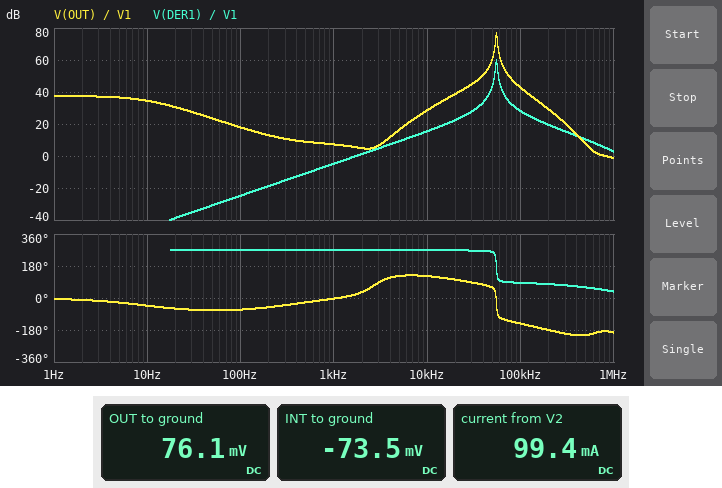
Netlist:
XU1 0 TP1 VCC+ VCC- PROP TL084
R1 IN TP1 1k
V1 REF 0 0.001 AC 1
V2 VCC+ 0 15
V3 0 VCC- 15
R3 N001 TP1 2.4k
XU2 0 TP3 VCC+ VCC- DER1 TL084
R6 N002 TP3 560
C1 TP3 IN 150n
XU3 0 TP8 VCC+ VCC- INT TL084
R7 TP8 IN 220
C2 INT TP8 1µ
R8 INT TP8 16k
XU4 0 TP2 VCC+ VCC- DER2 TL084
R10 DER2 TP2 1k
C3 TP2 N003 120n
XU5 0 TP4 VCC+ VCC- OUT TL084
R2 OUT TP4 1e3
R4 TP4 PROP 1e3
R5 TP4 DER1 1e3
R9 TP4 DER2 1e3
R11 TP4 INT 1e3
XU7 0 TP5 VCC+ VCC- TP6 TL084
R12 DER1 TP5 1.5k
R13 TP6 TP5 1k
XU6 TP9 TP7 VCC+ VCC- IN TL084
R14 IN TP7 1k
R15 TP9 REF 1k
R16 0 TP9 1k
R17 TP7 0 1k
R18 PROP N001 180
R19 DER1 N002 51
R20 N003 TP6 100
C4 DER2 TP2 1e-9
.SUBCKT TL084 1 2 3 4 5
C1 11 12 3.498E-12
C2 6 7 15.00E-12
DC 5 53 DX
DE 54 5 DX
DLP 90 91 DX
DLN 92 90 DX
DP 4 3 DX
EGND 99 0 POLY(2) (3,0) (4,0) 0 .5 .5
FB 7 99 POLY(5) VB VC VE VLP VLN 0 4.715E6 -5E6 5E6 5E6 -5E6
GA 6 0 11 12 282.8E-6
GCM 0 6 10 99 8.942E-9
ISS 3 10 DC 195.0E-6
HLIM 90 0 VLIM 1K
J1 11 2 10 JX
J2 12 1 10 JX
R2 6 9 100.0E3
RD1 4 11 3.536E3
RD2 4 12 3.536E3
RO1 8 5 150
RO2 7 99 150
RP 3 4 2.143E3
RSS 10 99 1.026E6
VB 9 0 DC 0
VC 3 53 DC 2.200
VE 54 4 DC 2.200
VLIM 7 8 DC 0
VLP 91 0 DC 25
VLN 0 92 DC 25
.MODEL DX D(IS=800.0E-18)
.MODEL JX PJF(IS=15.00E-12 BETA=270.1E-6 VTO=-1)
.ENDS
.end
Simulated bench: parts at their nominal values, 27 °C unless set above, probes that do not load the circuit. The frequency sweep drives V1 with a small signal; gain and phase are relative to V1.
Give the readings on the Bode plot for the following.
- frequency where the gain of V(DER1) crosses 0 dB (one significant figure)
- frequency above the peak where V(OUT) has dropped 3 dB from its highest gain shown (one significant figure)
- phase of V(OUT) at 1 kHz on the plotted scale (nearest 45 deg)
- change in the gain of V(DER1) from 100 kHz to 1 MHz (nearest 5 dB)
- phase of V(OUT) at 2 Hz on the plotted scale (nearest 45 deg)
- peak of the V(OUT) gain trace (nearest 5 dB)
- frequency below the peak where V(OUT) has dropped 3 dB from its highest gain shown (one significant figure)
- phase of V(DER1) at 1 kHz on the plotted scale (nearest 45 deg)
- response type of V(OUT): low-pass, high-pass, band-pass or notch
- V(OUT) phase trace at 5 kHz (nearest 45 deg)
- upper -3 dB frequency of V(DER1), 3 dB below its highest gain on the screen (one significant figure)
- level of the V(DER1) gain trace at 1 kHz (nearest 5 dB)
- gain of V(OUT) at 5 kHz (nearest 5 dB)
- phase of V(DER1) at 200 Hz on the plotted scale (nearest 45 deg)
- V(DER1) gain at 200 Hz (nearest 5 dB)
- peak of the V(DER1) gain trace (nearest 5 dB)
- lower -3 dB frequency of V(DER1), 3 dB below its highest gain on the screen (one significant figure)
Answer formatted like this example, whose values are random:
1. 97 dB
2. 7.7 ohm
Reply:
1. 2 kHz
2. 60 kHz
3. 0 deg
4. -25 dB
5. 0 deg
6. 75 dB
7. 50 kHz
8. 270 deg
9. band-pass
10. 135 deg
11. 60 kHz
12. -5 dB
13. 15 dB
14. 270 deg
15. -20 dB
16. 60 dB
17. 50 kHz
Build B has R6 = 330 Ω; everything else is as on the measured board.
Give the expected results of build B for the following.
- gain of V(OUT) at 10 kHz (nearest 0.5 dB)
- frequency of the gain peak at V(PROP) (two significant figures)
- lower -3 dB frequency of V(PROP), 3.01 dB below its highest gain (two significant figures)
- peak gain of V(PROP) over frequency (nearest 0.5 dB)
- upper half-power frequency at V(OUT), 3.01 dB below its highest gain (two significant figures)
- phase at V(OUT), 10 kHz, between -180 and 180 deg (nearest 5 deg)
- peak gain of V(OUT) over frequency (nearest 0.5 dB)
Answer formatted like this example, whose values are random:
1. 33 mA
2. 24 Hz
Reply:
1. 24.0 dB
2. 63 kHz
3. 62 kHz
4. 27.0 dB
5. 64 kHz
6. 120 deg
7. 72.0 dB
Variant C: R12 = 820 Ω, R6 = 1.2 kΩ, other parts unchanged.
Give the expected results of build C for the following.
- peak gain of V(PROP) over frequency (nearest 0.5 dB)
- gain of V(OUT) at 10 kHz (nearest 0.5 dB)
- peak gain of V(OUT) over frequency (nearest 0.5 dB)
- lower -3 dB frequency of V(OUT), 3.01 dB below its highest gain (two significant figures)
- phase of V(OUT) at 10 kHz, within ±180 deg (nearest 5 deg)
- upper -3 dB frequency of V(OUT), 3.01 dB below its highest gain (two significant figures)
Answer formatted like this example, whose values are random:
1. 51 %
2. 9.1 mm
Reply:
1. 21.0 dB
2. 40.0 dB
3. 85.0 dB
4. 41 kHz
5. 130 deg
6. 42 kHz
